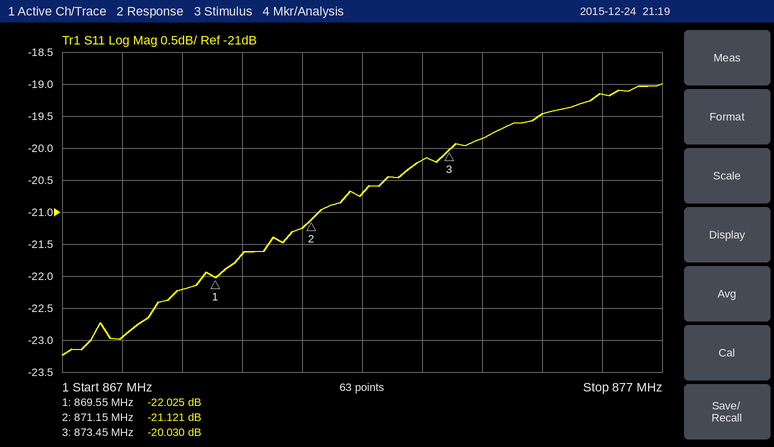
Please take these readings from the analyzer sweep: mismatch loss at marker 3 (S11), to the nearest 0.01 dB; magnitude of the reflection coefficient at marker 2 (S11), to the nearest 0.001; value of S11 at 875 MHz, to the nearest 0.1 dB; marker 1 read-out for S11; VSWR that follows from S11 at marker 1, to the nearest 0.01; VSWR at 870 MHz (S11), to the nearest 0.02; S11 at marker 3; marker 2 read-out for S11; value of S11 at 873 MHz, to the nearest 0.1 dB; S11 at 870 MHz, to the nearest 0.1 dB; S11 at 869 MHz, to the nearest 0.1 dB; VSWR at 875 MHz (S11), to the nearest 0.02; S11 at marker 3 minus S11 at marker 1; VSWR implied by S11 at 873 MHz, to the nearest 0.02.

0.04 dB
0.088
-19.5 dB
-22.025 dB
1.17
1.18
-20.030 dB
-21.121 dB
-20.2 dB
-21.7 dB
-22.2 dB
1.24
1.995 dB
1.22
